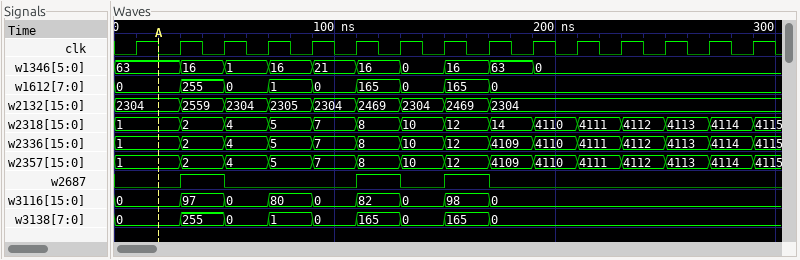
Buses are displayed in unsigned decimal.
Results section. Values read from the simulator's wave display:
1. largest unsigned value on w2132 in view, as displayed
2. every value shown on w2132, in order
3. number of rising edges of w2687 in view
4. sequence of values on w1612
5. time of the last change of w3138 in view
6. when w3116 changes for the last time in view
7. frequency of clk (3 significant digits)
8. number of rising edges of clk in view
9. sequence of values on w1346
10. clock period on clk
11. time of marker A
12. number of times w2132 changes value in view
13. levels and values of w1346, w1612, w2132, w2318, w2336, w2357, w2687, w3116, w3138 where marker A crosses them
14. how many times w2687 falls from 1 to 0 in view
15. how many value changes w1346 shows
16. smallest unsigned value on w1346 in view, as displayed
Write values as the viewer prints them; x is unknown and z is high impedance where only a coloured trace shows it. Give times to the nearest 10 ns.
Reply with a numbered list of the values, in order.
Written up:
1. 2559
2. 2304, 2559, 2304, 2305, 2304, 2469, 2304, 2469, 2304
3. 3
4. 0, 255, 0, 1, 0, 165, 0, 165, 0
5. 170 ns
6. 170 ns
7. 50.0 MHz
8. 15
9. 63, 16, 1, 16, 21, 16, 0, 16, 63, 0
10. 20 ns
11. 20 ns
12. 8
13. w1346=63, w1612=0, w2132=2304, w2318=1, w2336=1, w2357=1, w2687=0, w3116=0, w3138=0
14. 3
15. 9
16. 0
